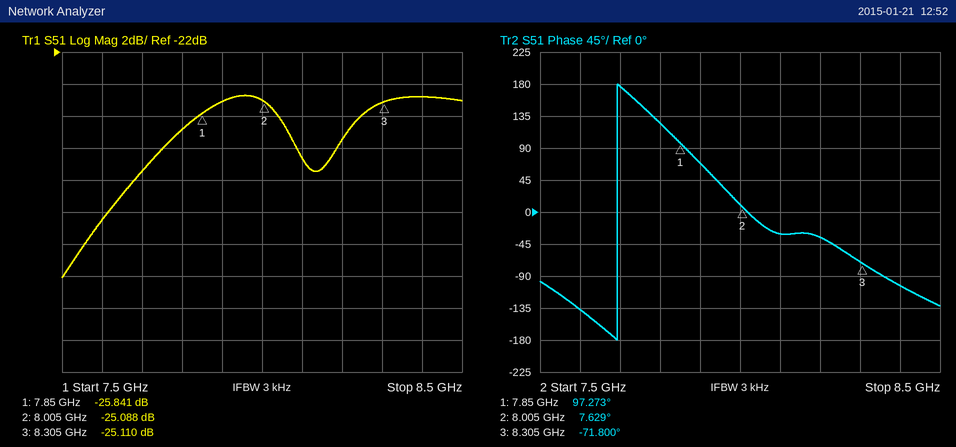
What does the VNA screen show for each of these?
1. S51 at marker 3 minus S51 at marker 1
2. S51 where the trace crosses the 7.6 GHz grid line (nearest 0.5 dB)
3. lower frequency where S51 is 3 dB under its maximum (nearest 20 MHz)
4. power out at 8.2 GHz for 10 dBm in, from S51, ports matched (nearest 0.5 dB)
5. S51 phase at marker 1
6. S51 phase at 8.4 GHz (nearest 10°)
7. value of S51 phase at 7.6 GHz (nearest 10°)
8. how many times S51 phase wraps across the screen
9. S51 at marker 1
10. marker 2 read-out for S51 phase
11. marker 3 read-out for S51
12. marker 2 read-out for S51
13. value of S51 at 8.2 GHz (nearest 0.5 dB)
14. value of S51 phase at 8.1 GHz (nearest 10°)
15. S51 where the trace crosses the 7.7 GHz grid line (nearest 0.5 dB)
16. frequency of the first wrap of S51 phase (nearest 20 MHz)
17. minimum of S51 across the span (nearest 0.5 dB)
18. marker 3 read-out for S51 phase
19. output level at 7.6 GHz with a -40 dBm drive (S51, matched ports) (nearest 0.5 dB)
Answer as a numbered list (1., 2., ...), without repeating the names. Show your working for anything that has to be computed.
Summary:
1. -25.11 − (-25.841) = 0.731 dB
2. -32.5 dB
3. 7.76 GHz
4. 10 dBm + (-27.5 dB) = -17.5 dBm
5. 97.273°
6. -100°
7. -140°
8. 1
9. -25.841 dB
10. 7.629°
11. -25.110 dB
12. -25.088 dB
13. -27.5 dB
14. -30°
15. -29.5 dB
16. 7.70 GHz
17. -36.0 dB
18. -71.800°
19. -40 dBm + (-32.5 dB) = -72.5 dBm
